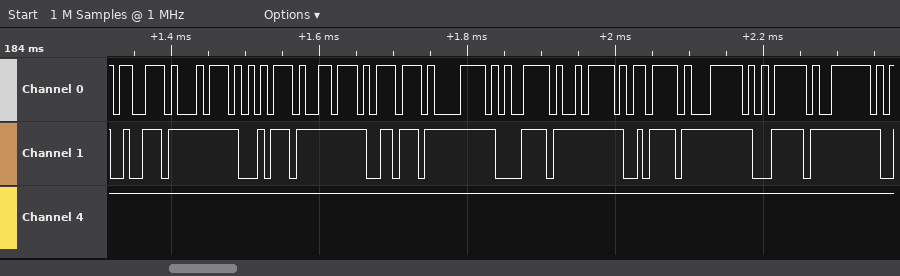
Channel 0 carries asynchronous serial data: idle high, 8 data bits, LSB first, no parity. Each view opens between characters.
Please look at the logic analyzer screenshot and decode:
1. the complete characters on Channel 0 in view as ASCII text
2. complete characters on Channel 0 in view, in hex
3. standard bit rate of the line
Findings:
"stuvwxyz{|}~"
73, 74, 75, 76, 77, 78, 79, 7A, 7B, 7C, 7D, 7E
115200 baud
